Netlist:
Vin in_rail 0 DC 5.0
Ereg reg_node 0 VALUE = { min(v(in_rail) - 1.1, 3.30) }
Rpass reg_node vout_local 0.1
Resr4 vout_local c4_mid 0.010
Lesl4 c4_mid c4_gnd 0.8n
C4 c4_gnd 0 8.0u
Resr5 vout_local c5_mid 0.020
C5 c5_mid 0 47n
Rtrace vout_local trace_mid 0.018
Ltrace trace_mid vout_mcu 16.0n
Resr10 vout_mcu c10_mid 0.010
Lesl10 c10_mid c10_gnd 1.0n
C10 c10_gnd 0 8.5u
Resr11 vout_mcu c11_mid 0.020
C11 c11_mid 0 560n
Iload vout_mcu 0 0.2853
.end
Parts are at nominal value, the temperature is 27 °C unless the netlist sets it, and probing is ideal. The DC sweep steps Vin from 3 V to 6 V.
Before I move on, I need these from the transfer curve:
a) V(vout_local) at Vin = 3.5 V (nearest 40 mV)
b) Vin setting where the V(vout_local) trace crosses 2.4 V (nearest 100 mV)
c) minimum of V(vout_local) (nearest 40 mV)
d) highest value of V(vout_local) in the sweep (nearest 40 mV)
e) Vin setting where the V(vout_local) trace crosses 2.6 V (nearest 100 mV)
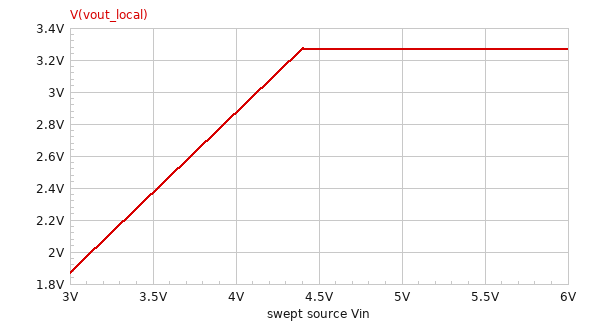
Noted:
2.36 V
3.5 V
1.88 V
3.28 V
3.7 V
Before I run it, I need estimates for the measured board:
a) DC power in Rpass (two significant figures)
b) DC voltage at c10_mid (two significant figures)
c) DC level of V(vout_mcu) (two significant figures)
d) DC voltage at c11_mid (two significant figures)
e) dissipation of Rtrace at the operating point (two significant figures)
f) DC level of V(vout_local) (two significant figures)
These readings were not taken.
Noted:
8.1 mW
3.3 V
3.3 V
3.3 V
1.5 mW
3.3 V
